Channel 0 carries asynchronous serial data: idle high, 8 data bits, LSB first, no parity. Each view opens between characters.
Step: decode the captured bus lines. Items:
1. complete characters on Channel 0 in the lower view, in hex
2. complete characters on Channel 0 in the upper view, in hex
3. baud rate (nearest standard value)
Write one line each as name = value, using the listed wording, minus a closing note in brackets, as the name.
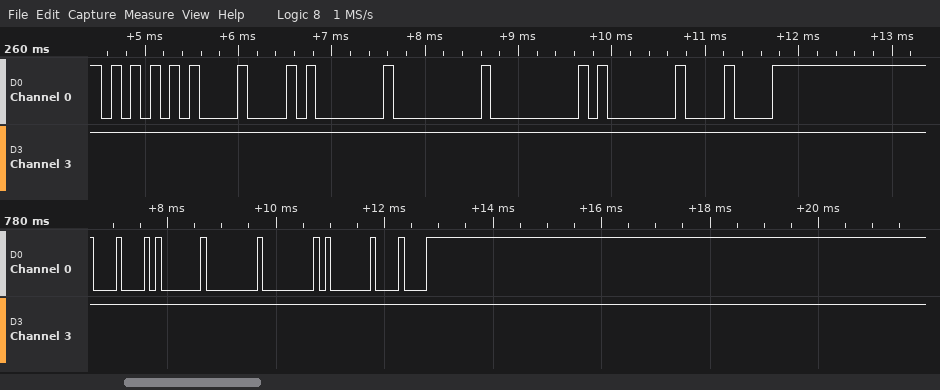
complete characters on Channel 0 in the lower view, in hex = 08, 01, 00, 00, 01, 08
complete characters on Channel 0 in the upper view, in hex = 55, 08, 01, 00, 00, 01, 08
baud rate = 9600 baud
